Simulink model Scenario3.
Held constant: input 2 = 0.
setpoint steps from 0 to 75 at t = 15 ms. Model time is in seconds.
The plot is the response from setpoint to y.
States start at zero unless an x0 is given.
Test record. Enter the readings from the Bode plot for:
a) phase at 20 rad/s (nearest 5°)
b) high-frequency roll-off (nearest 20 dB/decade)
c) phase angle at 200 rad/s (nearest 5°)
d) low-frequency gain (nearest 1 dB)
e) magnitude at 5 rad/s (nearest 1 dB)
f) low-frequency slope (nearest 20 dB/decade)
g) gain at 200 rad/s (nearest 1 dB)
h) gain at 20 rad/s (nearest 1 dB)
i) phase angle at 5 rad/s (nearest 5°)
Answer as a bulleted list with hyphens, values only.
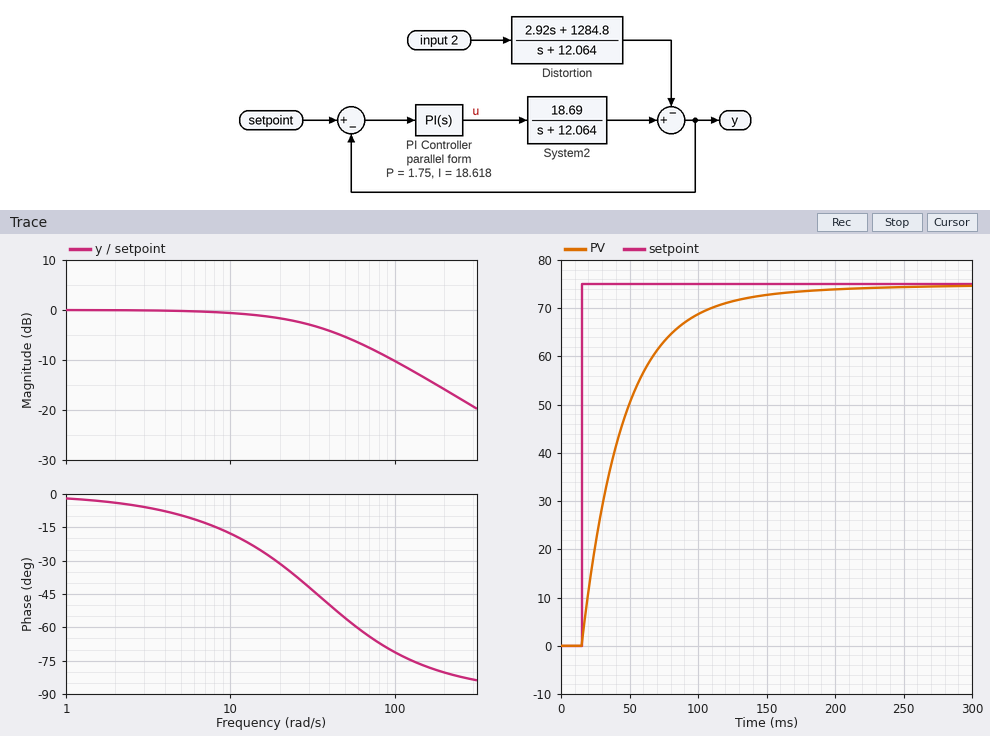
- -30°
- -20 dB/decade
- -80°
- 0 dB
- 0 dB
- 0 dB/decade
- -16 dB
- -2 dB
- -10°
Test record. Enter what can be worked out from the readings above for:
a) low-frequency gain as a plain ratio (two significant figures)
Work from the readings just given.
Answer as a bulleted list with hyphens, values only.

- 1.0
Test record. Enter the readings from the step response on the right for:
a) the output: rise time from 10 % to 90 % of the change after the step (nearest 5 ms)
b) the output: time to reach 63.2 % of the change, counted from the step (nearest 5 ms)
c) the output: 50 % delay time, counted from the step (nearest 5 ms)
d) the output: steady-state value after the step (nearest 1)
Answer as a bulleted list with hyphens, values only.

- 75 ms
- 30 ms
- 20 ms
- 75
